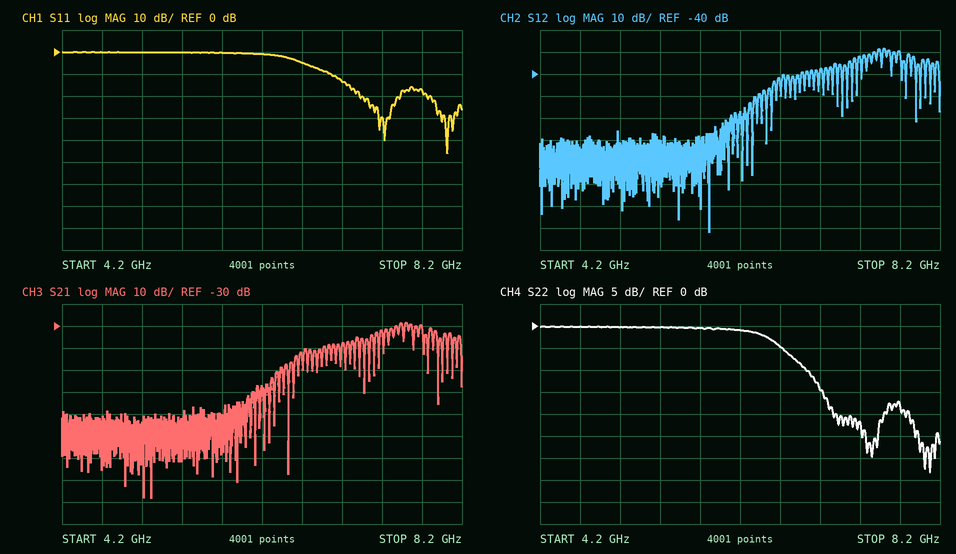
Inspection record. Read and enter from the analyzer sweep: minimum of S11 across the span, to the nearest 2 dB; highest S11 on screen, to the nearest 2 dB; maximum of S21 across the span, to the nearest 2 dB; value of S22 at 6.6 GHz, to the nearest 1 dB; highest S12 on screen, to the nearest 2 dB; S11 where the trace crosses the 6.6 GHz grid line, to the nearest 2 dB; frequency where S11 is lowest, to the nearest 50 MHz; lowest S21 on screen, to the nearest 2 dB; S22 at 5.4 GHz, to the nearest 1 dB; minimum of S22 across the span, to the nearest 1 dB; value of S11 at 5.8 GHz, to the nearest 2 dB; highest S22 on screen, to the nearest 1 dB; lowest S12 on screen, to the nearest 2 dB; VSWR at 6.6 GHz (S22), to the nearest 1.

-46 dB
0 dB
-28 dB
-5 dB
-28 dB
-4 dB
8.05 GHz
-108 dB
0 dB
-33 dB
0 dB
0 dB
-112 dB
4
